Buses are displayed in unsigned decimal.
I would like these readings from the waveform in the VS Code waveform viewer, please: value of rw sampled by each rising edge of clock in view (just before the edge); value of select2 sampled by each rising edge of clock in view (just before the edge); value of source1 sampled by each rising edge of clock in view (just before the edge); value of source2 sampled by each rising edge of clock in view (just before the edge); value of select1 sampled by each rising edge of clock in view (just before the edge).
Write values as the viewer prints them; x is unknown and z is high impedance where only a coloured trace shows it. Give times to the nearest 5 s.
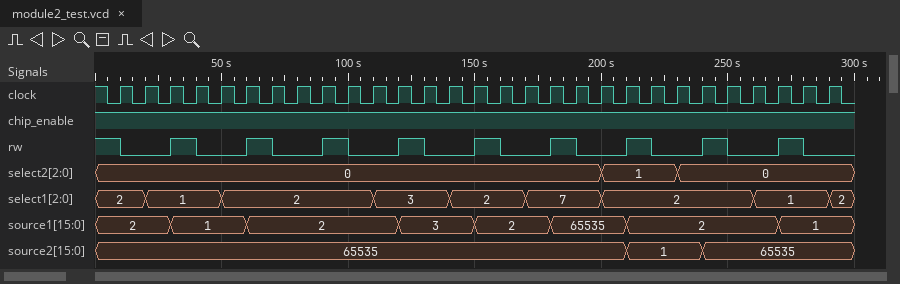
1 0 0 1 0 0 1 0 0 1 0 0 1 0 0 1 0 0 1 0 0 1 0 0 1 0 0 1 0
0, 0, 0, 0, 0, 0, 0, 0, 0, 0, 0, 0, 0, 0, 0, 0, 0, 0, 0, 0, 1, 1, 1, 0, 0, 0, 0, 0, 0
2, 2, 2, 1, 1, 1, 2, 2, 2, 2, 2, 2, 3, 3, 3, 2, 2, 2, 65535, 65535, 65535, 2, 2, 2, 2, 2, 2, 1, 1
65535, 65535, 65535, 65535, 65535, 65535, 65535, 65535, 65535, 65535, 65535, 65535, 65535, 65535, 65535, 65535, 65535, 65535, 65535, 65535, 65535, 1, 1, 1, 65535, 65535, 65535, 65535, 65535
2, 2, 1, 1, 1, 2, 2, 2, 2, 2, 2, 3, 3, 3, 2, 2, 2, 7, 7, 7, 2, 2, 2, 2, 2, 2, 1, 1, 1
